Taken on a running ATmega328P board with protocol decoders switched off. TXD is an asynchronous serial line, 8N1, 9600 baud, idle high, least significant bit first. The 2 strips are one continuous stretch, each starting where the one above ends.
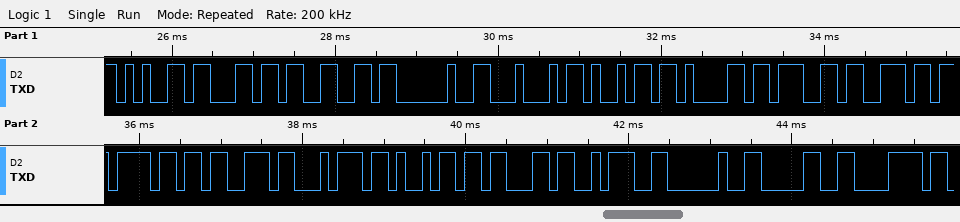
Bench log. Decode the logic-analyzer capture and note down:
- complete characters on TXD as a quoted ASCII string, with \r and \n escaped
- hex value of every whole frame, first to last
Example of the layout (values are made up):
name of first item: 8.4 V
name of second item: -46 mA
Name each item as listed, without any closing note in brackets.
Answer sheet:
complete characters on TXD as a quoted ASCII string, with \r and \n escaped: "elf Diagnostic: 0x"
hex value of every whole frame, first to last: 0x65 0x6C 0x66 0x20 0x44 0x69 0x61 0x67 0x6E 0x6F 0x73 0x74 0x69 0x63 0x3A 0x20 0x30 0x78
